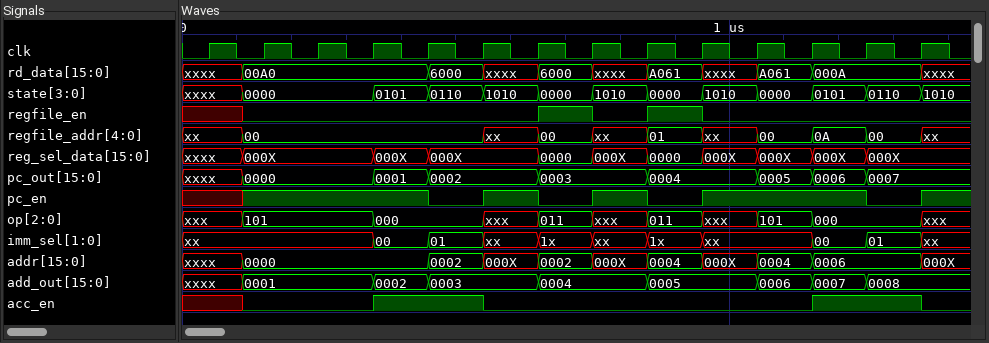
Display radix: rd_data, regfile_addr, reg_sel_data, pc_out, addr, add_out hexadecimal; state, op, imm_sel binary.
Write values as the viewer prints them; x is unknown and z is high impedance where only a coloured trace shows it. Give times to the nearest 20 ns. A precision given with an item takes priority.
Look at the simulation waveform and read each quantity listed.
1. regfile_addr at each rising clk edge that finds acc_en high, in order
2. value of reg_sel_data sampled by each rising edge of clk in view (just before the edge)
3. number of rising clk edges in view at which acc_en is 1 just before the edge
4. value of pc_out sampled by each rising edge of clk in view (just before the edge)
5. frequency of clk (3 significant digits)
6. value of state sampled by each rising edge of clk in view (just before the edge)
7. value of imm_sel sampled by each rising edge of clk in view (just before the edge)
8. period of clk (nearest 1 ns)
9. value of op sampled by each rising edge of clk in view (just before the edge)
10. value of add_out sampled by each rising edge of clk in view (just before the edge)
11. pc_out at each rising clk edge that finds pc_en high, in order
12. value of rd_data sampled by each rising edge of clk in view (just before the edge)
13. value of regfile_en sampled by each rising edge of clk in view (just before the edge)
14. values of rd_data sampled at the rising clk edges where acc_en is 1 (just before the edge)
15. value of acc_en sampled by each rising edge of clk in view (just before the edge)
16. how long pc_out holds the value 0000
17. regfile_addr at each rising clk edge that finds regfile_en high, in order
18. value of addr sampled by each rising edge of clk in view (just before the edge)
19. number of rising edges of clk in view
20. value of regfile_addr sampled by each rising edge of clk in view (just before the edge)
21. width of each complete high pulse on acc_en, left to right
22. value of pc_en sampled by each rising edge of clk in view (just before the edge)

00, 00, 0A, 00
xxxx, 000X, 000X, 000X, 000X, 000X, 000X, 0000, 000X, 0000, 000X, 000X, 000X, 000X
4
xxxx, 0000, 0000, 0000, 0001, 0002, 0002, 0003, 0003, 0004, 0004, 0005, 0006, 0007
10.0 MHz
xxxx, 0000, 0000, 0000, 0101, 0110, 1010, 0000, 1010, 0000, 1010, 0000, 0101, 0110
xx, xx, xx, xx, 00, 01, xx, 1x, xx, 1x, xx, xx, 00, 01
100 ns
xxx, 101, 101, 101, 000, 000, xxx, 011, xxx, 011, xxx, 101, 000, 000
xxxx, 0001, 0001, 0001, 0002, 0003, 0003, 0004, 0004, 0005, 0005, 0006, 0007, 0008
0000, 0000, 0000, 0001, 0002, 0003, 0004, 0005, 0006
xxxx, 00A0, 00A0, 00A0, 00A0, 6000, xxxx, 6000, xxxx, A061, xxxx, A061, 000A, 000A
x 0 0 0 0 0 0 1 0 1 0 0 0 0
00A0, 6000, 000A, 000A
x 0 0 0 1 1 0 0 0 0 0 0 1 1
240 ns
00, 01
xxxx, 0000, 0000, 0000, 0000, 0002, 000X, 0002, 000X, 0004, 000X, 0004, 0006, 0006
14
xx, 00, 00, 00, 00, 00, xx, 00, xx, 01, xx, 00, 0A, 00
200 ns, 200 ns
x 1 1 1 1 0 1 0 1 0 1 1 1 0
